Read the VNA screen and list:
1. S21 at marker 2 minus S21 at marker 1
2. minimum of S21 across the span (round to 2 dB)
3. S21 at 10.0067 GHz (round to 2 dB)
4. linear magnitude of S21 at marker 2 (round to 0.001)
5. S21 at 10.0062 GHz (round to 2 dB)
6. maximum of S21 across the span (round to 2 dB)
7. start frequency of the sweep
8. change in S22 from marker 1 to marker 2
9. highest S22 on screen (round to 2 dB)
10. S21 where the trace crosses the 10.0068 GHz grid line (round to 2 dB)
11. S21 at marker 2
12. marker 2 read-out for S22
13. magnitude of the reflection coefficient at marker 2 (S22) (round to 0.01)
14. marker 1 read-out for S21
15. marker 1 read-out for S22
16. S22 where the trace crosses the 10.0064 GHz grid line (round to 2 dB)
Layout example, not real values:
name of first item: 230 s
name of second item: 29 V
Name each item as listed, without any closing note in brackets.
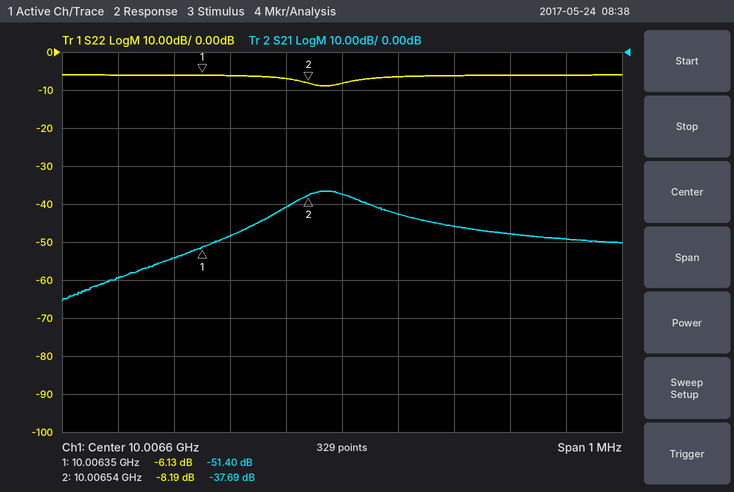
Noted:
S21 at marker 2 minus S21 at marker 1: 13.71 dB
minimum of S21 across the span: -66 dB
S21 at 10.0067 GHz: -42 dB
linear magnitude of S21 at marker 2: 0.013
S21 at 10.0062 GHz: -60 dB
maximum of S21 across the span: -36 dB
start frequency of the sweep: 10.0061 GHz
change in S22 from marker 1 to marker 2: -2.06 dB
highest S22 on screen: -6 dB
S21 where the trace crosses the 10.0068 GHz grid line: -46 dB
S21 at marker 2: -37.69 dB
marker 2 read-out for S22: -8.19 dB
magnitude of the reflection coefficient at marker 2 (S22): 0.39
marker 1 read-out for S21: -51.40 dB
marker 1 read-out for S22: -6.13 dB
S22 where the trace crosses the 10.0064 GHz grid line: -6 dB
